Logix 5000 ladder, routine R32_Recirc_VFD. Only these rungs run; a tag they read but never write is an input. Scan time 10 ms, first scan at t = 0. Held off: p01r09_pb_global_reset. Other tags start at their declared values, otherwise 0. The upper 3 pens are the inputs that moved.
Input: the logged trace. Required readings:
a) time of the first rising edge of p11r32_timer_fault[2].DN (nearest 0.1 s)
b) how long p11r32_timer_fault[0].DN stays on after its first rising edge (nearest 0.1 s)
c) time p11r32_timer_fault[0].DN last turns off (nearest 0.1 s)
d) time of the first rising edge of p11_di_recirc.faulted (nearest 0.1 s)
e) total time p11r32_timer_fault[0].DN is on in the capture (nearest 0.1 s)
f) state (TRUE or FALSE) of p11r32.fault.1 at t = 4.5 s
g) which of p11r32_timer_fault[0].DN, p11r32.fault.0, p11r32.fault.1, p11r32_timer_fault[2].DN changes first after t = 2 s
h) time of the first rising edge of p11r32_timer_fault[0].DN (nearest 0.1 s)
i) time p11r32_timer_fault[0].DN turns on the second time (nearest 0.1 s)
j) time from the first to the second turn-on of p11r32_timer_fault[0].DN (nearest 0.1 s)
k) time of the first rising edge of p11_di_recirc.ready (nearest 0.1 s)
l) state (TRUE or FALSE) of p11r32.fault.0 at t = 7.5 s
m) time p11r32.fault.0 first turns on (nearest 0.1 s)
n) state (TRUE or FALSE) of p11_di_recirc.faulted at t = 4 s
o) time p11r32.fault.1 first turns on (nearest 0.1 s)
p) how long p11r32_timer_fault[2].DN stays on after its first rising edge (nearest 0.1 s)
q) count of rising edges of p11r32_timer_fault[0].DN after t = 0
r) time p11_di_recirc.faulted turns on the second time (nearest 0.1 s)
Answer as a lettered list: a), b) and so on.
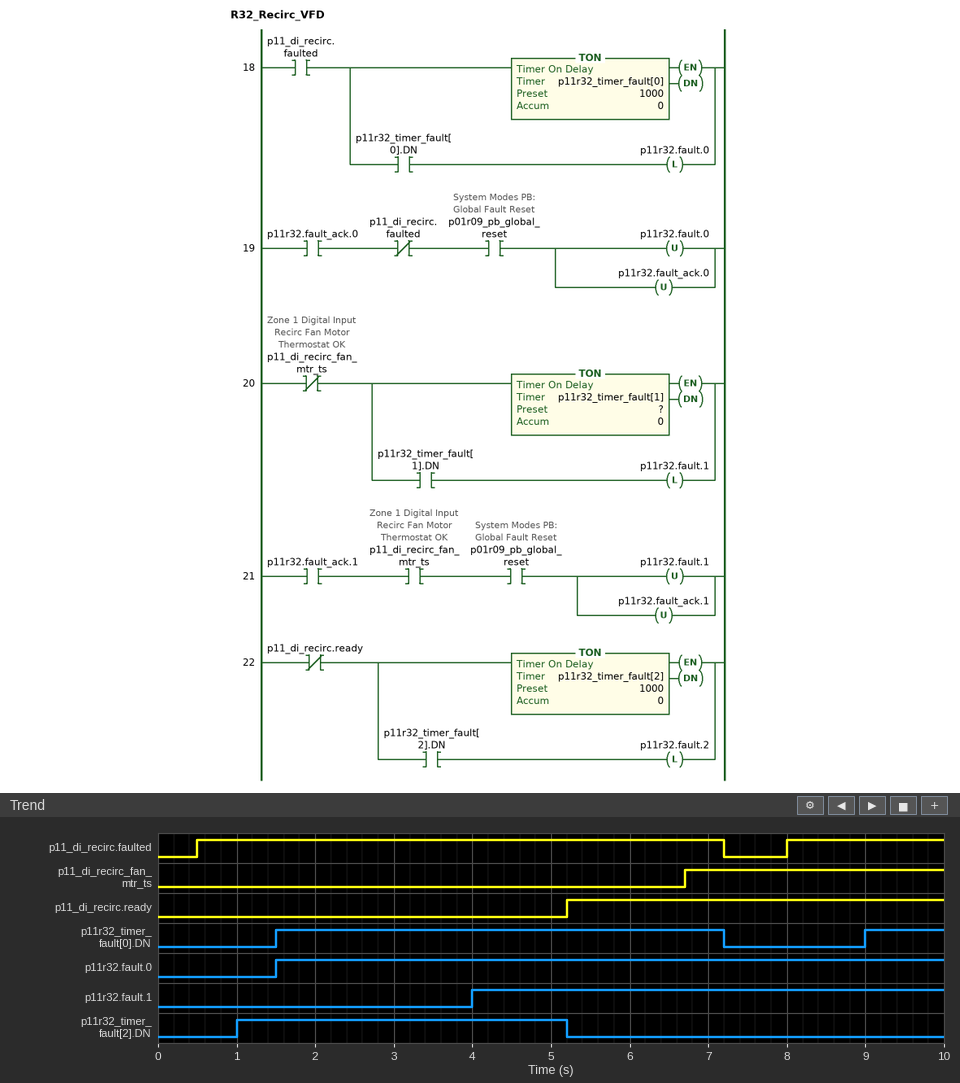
a) 1.0 s
b) 5.7 s
c) 7.2 s
d) 0.5 s
e) 6.7 s
f) TRUE
g) p11r32.fault.1
h) 1.5 s
i) 9.0 s
j) 7.5 s
k) 5.2 s
l) TRUE
m) 1.5 s
n) TRUE
o) 4.0 s
p) 4.2 s
q) 2
r) 8.0 s
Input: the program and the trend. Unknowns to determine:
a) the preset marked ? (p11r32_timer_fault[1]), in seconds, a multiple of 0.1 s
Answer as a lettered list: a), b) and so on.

a) 4.0 s
